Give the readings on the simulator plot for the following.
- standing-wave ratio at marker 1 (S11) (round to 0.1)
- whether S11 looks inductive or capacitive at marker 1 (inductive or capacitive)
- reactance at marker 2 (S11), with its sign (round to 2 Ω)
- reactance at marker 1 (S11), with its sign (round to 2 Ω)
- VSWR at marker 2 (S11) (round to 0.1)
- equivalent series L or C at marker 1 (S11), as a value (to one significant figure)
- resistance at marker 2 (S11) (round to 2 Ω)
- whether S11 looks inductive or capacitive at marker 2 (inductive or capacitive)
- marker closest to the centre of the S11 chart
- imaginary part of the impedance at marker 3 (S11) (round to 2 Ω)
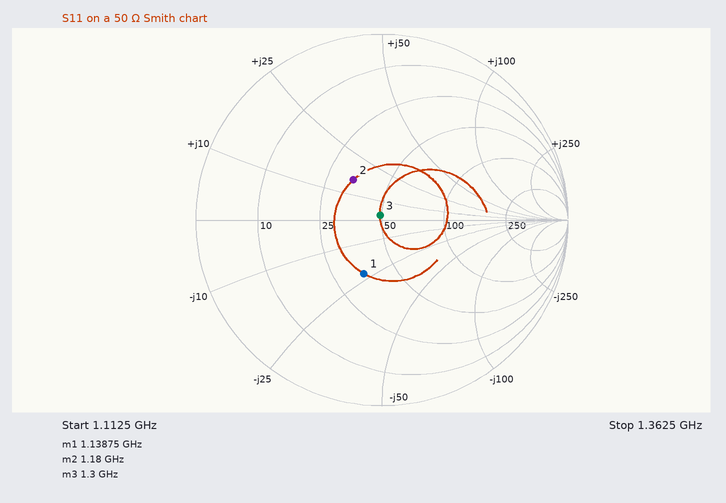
1.9
capacitive
+16 Ω
-22 Ω
1.7
6 pF
34 Ω
inductive
marker 3
+2 Ω
